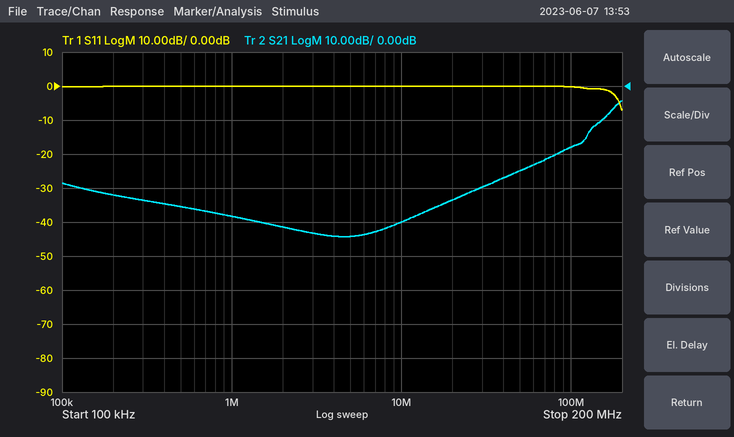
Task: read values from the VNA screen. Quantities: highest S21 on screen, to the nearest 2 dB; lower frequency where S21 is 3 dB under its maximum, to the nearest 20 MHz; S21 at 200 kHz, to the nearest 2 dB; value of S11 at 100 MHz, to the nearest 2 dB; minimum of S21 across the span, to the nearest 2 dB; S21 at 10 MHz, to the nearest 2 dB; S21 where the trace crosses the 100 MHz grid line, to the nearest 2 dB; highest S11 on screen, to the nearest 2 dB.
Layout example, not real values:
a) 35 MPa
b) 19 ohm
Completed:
a) -4 dB
b) 180 MHz
c) -32 dB
d) 0 dB
e) -44 dB
f) -40 dB
g) -18 dB
h) 0 dB
